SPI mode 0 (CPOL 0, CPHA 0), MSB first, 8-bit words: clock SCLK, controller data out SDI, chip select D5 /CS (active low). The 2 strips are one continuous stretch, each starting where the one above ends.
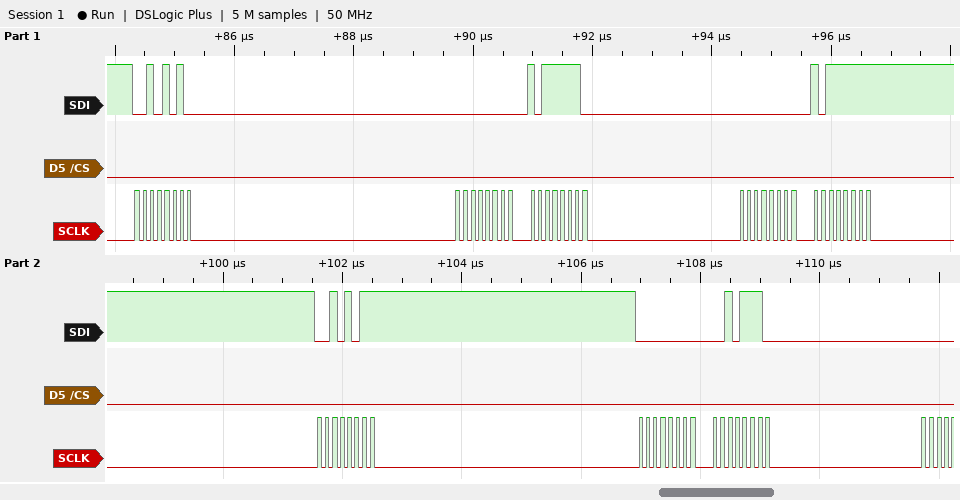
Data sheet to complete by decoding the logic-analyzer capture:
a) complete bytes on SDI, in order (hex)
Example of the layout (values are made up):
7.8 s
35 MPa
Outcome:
2A 00 BE 00 BF 2B 00 2E
